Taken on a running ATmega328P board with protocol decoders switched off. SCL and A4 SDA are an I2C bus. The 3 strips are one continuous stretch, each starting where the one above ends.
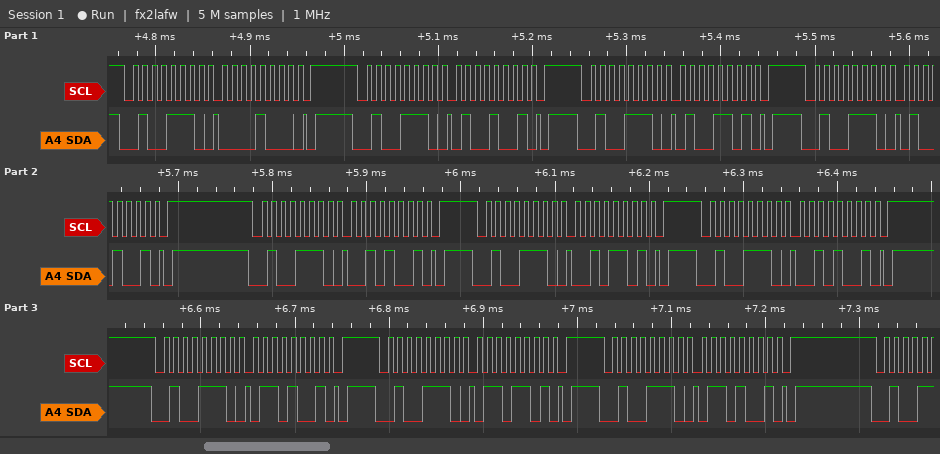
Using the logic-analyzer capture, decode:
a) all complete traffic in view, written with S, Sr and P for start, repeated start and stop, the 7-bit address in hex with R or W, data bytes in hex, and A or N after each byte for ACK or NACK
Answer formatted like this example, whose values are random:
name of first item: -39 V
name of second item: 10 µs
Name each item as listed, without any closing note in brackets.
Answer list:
all complete traffic in view, written with S, Sr and P for start, repeated start and stop, the 7-bit address in hex with R or W, data bytes in hex, and A or N after each byte for ACK or NACK: S 27W A 08 A P S 27W A 49 A P S 27W A 4D A P S 27W A 49 A P S 27W A 29 A P S 27W A 2D A P S 27W A 29 A P S 27W A 69 A P S 27W A 6D A P S 27W A 69 A P
